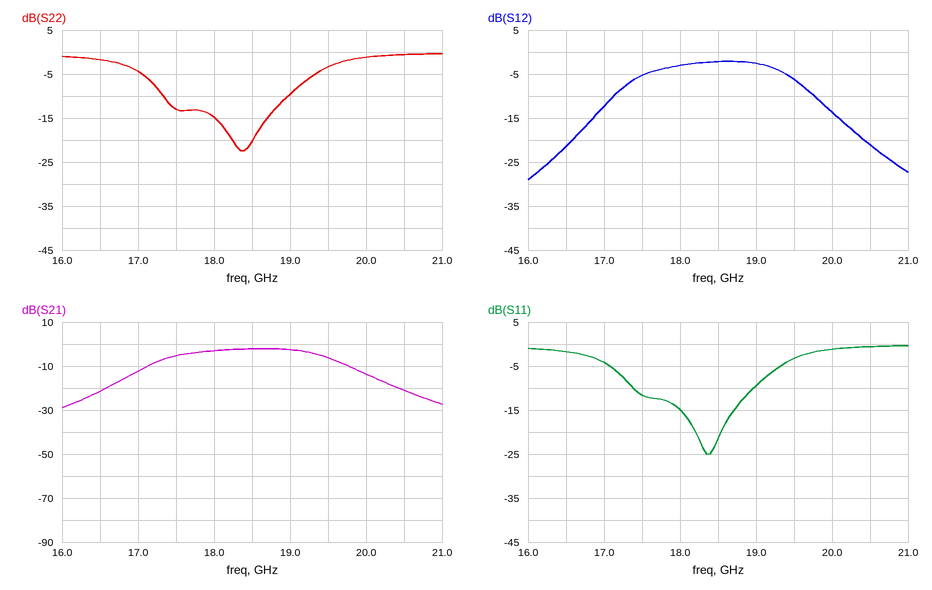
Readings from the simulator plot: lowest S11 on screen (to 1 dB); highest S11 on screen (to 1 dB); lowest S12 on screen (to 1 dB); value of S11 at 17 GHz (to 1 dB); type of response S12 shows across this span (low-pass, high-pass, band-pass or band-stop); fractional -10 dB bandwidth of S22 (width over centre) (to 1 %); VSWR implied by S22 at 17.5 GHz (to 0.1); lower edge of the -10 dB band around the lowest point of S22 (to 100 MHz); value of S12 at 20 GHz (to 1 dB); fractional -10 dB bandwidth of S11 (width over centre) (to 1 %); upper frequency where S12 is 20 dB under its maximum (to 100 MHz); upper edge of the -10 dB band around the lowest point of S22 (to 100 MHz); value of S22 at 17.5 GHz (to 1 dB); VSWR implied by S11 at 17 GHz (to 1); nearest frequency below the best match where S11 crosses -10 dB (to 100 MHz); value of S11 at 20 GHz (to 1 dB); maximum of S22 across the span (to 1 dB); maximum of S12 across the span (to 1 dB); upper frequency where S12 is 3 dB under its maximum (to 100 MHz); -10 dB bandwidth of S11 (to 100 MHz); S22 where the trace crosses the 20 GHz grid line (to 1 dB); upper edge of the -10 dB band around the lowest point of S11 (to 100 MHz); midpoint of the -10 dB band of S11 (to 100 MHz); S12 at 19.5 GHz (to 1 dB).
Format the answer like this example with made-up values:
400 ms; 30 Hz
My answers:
-25 dB; 0 dB; -29 dB; -4 dB; band-pass; 9 %; 1.6; 17.3 GHz; -14 dB; 9 %; 20.6 GHz; 19.0 GHz; -13 dB; 4; 17.4 GHz; -1 dB; 0 dB; -2 dB; 19.4 GHz; 1.6 GHz; -1 dB; 19.0 GHz; 18.2 GHz; -6 dB
